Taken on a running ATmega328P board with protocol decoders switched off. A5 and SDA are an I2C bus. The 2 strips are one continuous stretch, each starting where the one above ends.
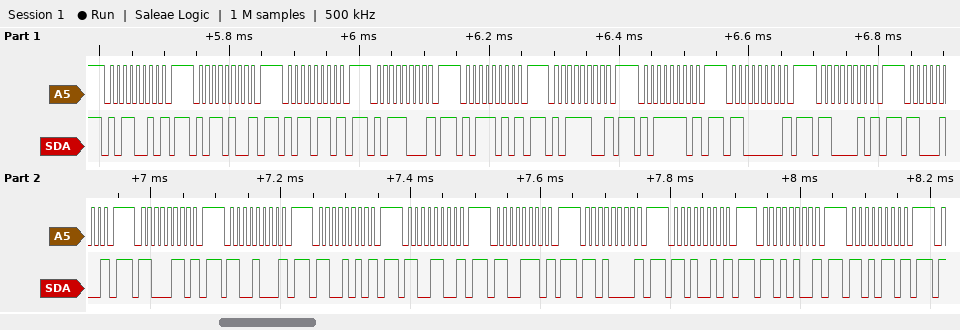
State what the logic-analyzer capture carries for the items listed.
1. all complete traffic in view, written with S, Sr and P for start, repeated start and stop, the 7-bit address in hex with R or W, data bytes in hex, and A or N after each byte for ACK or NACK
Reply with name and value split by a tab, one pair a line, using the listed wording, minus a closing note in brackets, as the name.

all complete traffic in view, written with S, Sr and P for start, repeated start and stop, the 7-bit address in hex with R or W, data bytes in hex, and A or N after each byte for ACK or NACK	S 59W N P S 5AW N P S 5BW N P S 5CW N P S 5DW N P S 5EW N P S 5FW N P S 60W N P S 61W N P S 62W N P S 63W N P S 64W N P S 65W N P S 66W N P S 67W N P S 68W N P S 69W N P S 6AW N P S 6BW N P
